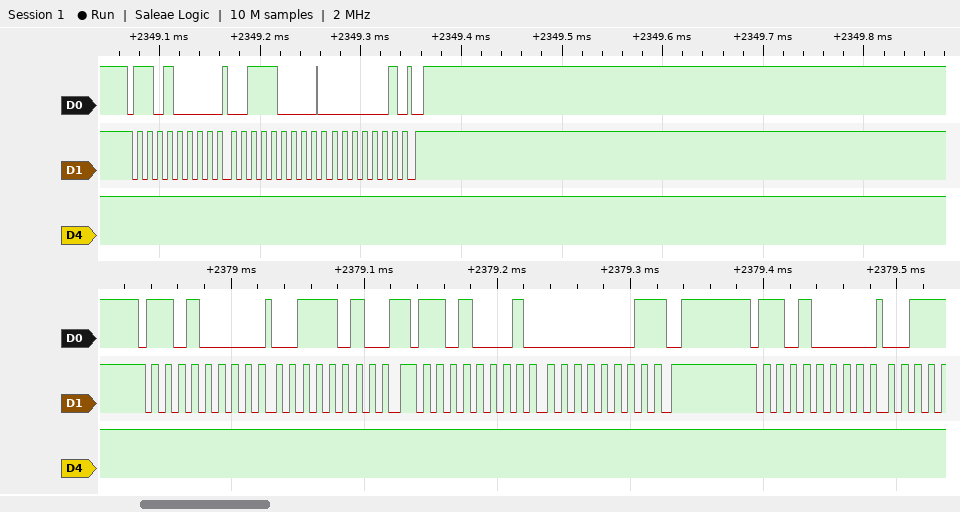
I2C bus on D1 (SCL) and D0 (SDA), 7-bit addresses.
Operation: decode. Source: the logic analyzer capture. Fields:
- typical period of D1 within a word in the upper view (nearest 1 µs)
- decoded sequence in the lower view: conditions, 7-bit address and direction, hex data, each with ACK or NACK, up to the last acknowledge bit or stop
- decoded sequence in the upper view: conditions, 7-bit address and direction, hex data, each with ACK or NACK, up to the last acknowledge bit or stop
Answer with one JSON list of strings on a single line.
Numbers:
["10 µs", "start, address 68 write ACK, 3A ACK, repeated start, address 68 read ACK, 01 NACK, stop, start, address 68 write ACK", "start, address 68 write ACK, 38 ACK, 01 ACK, stop"]
